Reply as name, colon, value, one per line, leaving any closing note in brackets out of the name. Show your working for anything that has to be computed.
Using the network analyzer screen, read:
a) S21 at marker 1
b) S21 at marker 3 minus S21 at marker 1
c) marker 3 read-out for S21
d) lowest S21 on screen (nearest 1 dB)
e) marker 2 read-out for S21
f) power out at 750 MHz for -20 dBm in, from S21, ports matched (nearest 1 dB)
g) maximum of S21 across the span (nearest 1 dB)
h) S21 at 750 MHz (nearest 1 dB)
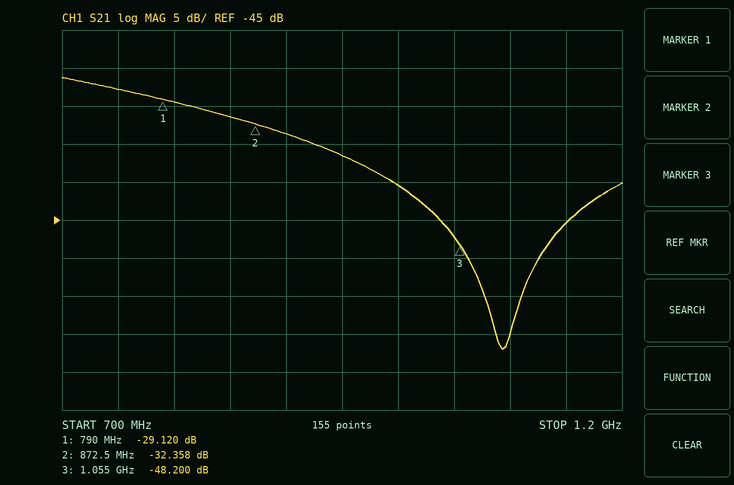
S21 at marker 1: -29.120 dB
S21 at marker 3 minus S21 at marker 1: -48.2 − (-29.12) = -19.080 dB
marker 3 read-out for S21: -48.200 dB
lowest S21 on screen: -62 dB
marker 2 read-out for S21: -32.358 dB
power out at 750 MHz for -20 dBm in, from S21, ports matched: -20 dBm + (-28 dB) = -48 dBm
maximum of S21 across the span: -26 dB
S21 at 750 MHz: -28 dB
